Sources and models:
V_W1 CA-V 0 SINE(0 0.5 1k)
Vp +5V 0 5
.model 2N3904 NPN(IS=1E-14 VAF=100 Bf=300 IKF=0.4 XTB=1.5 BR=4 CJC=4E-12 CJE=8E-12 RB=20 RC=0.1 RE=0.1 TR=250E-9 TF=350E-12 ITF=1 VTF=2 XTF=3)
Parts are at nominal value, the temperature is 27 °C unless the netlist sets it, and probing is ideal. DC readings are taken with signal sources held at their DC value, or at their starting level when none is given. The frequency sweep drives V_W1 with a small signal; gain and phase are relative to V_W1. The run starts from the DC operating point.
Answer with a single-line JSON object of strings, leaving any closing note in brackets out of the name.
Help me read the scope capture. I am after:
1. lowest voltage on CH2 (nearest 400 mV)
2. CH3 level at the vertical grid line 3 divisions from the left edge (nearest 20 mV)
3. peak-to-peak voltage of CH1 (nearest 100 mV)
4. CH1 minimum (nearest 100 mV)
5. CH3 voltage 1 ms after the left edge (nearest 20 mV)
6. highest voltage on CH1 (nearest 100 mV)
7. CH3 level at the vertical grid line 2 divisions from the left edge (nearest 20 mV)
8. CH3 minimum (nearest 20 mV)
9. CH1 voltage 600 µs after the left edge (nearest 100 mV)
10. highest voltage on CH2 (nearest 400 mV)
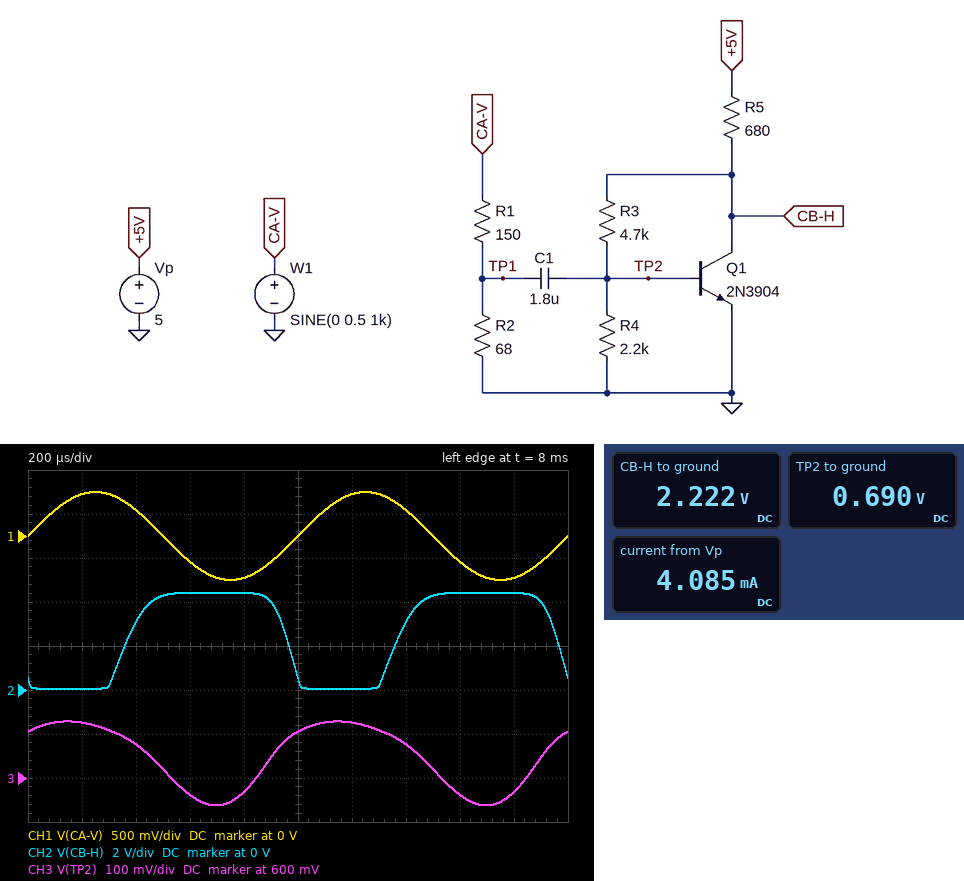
{"lowest voltage on CH2": "0 V", "CH3 level at the vertical grid line 3 divisions from the left edge": "560 mV", "peak-to-peak voltage of CH1": "1.0 V", "CH1 minimum": "-500 mV", "CH3 voltage 1 ms after the left edge": "700 mV", "highest voltage on CH1": "500 mV", "CH3 level at the vertical grid line 2 divisions from the left edge": "680 mV", "CH3 minimum": "540 mV", "CH1 voltage 600 µs after the left edge": "-300 mV", "highest voltage on CH2": "4.4 V"}
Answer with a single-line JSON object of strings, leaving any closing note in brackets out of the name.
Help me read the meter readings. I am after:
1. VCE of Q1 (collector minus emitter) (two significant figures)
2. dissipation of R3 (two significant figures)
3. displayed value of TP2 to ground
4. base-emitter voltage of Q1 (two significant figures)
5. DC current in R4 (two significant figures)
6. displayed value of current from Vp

{"VCE of Q1 (collector minus emitter)": "2.2 V", "dissipation of R3": "500 µW", "displayed value of TP2 to ground": "0.690 V", "base-emitter voltage of Q1": "690 mV", "DC current in R4": "310 µA", "displayed value of current from Vp": "4.085 mA"}
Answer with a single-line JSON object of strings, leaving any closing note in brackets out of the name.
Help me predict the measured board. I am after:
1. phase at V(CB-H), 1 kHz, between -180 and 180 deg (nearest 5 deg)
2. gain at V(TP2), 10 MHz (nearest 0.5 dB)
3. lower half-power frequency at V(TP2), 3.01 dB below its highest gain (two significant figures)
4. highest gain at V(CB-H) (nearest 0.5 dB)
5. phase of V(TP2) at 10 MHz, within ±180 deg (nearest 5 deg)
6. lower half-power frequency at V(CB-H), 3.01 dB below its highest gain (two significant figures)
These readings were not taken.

{"phase at V(CB-H), 1 kHz, between -180 and 180 deg": "-140 deg", "gain at V(TP2), 10 MHz": "-16.5 dB", "lower half-power frequency at V(TP2), 3.01 dB below its highest gain": "880 Hz", "highest gain at V(CB-H)": "22.5 dB", "phase of V(TP2) at 10 MHz, within ±180 deg": "-10 deg", "lower half-power frequency at V(CB-H), 3.01 dB below its highest gain": "880 Hz"}
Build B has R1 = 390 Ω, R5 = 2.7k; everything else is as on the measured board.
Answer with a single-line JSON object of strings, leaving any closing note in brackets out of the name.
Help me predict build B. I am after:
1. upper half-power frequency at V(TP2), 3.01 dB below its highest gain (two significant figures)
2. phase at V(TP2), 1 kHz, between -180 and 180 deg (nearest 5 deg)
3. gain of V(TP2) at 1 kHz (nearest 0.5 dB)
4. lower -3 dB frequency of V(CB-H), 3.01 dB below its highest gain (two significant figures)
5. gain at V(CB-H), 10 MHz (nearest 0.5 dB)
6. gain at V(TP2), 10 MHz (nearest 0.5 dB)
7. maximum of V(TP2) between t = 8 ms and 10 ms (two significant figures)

{"upper half-power frequency at V(TP2), 3.01 dB below its highest gain": "160 MHz", "phase at V(TP2), 1 kHz, between -180 and 180 deg": "30 deg", "gain of V(TP2) at 1 kHz": "-22.5 dB", "lower -3 dB frequency of V(CB-H), 3.01 dB below its highest gain": "620 Hz", "gain at V(CB-H), 10 MHz": "11.5 dB", "gain at V(TP2), 10 MHz": "-21.5 dB", "maximum of V(TP2) between t = 8 ms and 10 ms": "670 mV"}
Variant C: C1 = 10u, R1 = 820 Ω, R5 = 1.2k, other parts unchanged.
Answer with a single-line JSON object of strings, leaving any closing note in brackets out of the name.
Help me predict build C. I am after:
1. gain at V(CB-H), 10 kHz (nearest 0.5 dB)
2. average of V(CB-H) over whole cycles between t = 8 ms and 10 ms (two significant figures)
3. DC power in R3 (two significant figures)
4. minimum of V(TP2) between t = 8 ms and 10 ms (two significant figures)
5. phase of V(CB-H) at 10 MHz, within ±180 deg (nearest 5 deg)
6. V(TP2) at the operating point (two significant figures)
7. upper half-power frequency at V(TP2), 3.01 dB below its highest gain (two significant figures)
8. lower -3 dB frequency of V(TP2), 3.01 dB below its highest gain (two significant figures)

{"gain at V(CB-H), 10 kHz": "9.0 dB", "average of V(CB-H) over whole cycles between t = 8 ms and 10 ms": "2.1 V", "DC power in R3": "460 µW", "minimum of V(TP2) between t = 8 ms and 10 ms": "650 mV", "phase of V(CB-H) at 10 MHz, within ±180 deg": "145 deg", "V(TP2) at the operating point": "670 mV", "upper half-power frequency at V(TP2), 3.01 dB below its highest gain": "38 MHz", "lower -3 dB frequency of V(TP2), 3.01 dB below its highest gain": "130 Hz"}
